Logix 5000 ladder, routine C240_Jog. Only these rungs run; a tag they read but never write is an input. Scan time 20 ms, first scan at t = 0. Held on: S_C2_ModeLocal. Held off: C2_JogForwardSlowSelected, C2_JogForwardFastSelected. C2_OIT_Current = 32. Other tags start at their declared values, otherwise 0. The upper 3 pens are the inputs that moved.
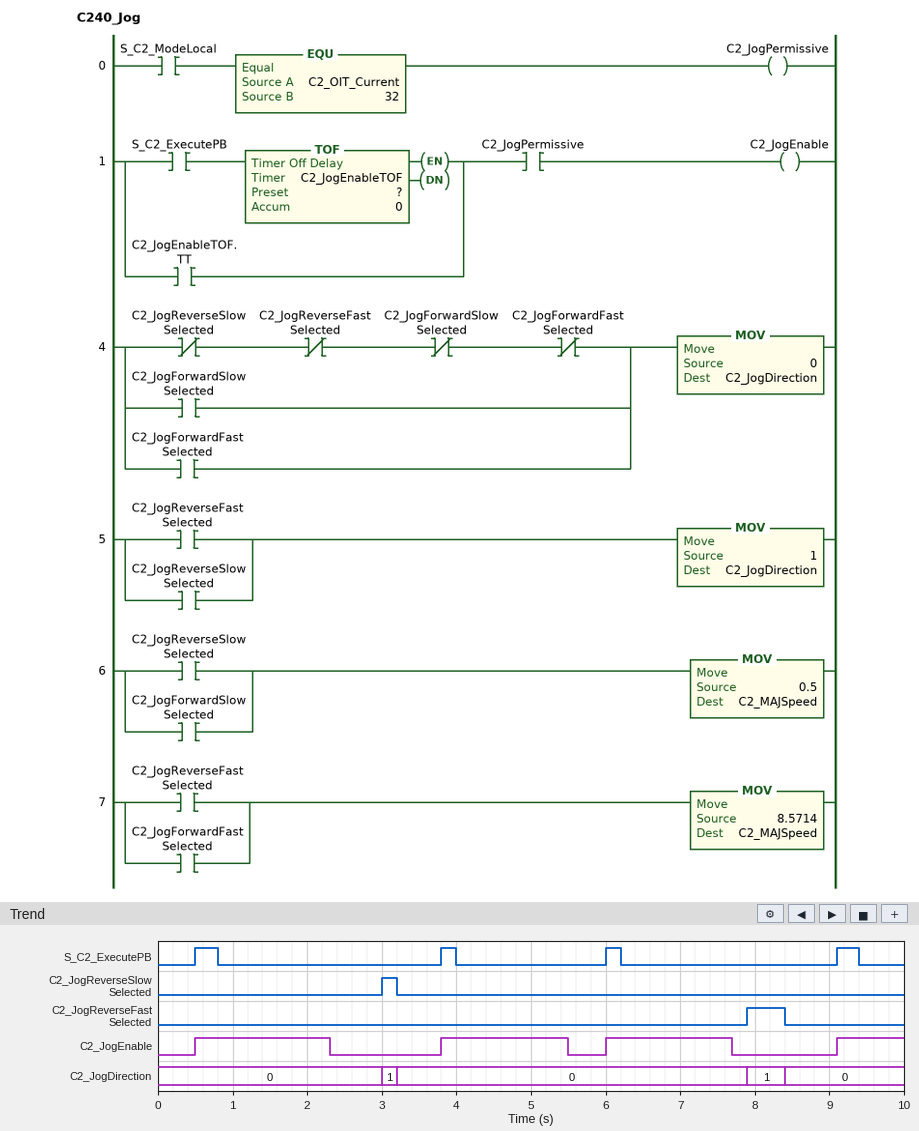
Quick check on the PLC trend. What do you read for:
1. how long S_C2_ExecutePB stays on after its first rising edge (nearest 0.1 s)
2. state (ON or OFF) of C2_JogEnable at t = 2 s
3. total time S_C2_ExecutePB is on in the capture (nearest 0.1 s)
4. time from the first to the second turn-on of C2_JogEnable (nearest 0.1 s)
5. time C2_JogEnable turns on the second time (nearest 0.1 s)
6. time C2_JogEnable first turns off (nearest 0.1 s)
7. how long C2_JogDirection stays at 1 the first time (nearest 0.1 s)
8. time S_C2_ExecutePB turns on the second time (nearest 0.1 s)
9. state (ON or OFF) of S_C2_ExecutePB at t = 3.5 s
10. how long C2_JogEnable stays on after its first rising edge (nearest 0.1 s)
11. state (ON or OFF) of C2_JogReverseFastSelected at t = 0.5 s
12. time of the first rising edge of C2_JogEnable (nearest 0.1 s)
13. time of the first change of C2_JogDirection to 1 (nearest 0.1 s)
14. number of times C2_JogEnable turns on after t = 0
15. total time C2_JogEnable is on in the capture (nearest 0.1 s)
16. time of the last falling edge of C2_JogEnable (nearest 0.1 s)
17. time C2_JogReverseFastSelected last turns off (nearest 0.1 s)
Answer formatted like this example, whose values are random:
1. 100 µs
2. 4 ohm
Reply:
1. 0.3 s
2. ON
3. 1.0 s
4. 3.3 s
5. 3.8 s
6. 2.3 s
7. 0.2 s
8. 3.8 s
9. OFF
10. 1.8 s
11. OFF
12. 0.5 s
13. 3.0 s
14. 4
15. 6.1 s
16. 7.7 s
17. 8.4 s
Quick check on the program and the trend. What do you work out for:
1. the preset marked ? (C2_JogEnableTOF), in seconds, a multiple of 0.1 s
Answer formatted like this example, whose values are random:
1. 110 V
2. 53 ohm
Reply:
1. 1.5 s
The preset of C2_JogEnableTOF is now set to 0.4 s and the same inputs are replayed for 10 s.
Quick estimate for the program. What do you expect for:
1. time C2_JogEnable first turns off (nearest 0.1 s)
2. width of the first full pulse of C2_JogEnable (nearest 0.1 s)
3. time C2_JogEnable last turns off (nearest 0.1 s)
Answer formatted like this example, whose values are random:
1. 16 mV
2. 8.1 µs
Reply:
1. 1.2 s
2. 0.7 s
3. 9.8 s
